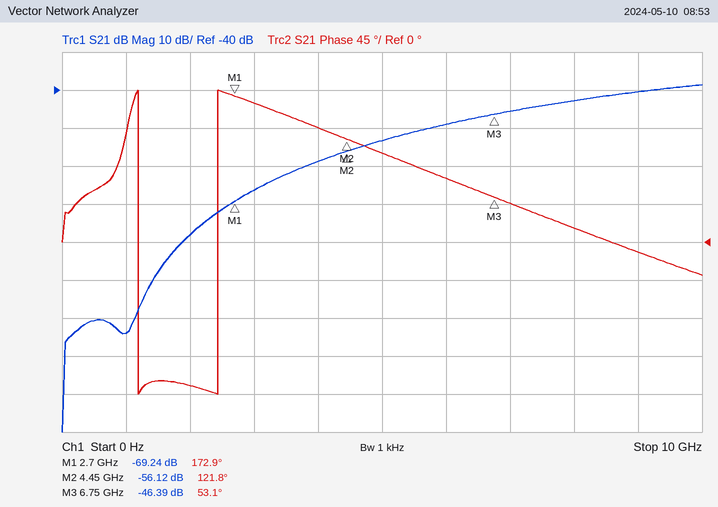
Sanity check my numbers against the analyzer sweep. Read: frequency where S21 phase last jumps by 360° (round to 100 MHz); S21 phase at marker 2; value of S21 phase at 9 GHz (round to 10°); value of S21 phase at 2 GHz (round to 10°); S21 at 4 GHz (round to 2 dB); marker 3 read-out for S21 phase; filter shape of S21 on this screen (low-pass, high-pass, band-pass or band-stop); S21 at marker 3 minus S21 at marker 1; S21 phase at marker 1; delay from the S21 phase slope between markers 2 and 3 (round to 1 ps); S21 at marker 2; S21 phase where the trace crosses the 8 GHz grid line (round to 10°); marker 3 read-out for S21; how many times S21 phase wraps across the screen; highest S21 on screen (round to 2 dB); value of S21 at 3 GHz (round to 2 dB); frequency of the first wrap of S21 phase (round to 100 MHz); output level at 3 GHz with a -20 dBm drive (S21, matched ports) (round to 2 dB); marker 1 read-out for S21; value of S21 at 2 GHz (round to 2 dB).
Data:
2.4 GHz
121.8°
-10°
-170°
-58 dB
53.1°
high-pass
22.85 dB
172.9°
83 ps
-56.12 dB
20°
-46.39 dB
2
-38 dB
-66 dB
1.2 GHz
-86 dBm
-69.24 dB
-78 dB
